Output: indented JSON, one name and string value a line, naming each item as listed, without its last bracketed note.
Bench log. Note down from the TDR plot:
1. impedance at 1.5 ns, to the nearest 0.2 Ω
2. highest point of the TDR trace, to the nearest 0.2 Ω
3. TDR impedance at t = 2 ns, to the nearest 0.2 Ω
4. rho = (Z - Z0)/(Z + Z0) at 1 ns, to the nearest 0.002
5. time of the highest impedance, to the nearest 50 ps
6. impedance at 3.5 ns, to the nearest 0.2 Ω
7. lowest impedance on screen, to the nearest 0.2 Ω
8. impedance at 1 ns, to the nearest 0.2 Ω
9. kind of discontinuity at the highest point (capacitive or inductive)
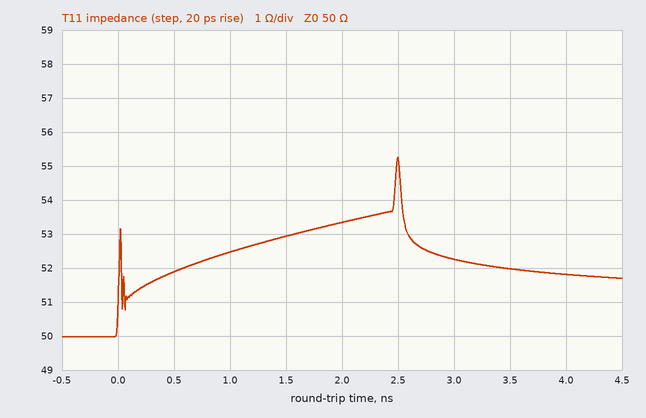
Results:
{
  "impedance at 1.5 ns, to the nearest 0.2 Ω": "53.0 Ω",
  "highest point of the TDR trace, to the nearest 0.2 Ω": "55.2 Ω",
  "TDR impedance at t = 2 ns, to the nearest 0.2 Ω": "53.4 Ω",
  "rho = (Z - Z0)/(Z + Z0) at 1 ns, to the nearest 0.002": "+0.024",
  "time of the highest impedance, to the nearest 50 ps": "2.50 ns",
  "impedance at 3.5 ns, to the nearest 0.2 Ω": "52.0 Ω",
  "lowest impedance on screen, to the nearest 0.2 Ω": "50.0 Ω",
  "impedance at 1 ns, to the nearest 0.2 Ω": "52.4 Ω",
  "kind of discontinuity at the highest point": "inductive"
}
